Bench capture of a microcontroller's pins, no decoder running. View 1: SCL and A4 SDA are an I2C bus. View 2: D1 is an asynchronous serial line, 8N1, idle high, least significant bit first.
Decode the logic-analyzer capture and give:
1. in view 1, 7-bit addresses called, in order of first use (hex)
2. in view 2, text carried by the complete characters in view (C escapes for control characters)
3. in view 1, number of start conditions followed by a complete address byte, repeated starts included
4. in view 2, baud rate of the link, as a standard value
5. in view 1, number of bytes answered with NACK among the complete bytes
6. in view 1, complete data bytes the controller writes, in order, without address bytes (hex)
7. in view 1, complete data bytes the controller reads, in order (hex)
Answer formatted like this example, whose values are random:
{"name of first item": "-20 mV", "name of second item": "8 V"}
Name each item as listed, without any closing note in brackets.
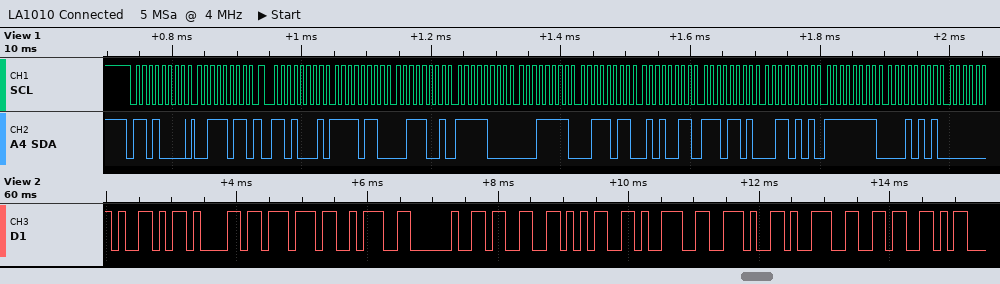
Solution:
{"in view 1, 7-bit addresses called, in order of first use": "0x68", "in view 2, text carried by the complete characters in view": "\"Yaw: 359.96\"", "in view 1, number of start conditions followed by a complete address byte, repeated starts included": "2", "in view 2, baud rate of the link, as a standard value": "9600 baud", "in view 1, number of bytes answered with NACK among the complete bytes": "0", "in view 1, complete data bytes the controller writes, in order, without address bytes": "3B", "in view 1, complete data bytes the controller reads, in order": "F6 39 F8 1F 3B 53 ED 35 FF 15"}
